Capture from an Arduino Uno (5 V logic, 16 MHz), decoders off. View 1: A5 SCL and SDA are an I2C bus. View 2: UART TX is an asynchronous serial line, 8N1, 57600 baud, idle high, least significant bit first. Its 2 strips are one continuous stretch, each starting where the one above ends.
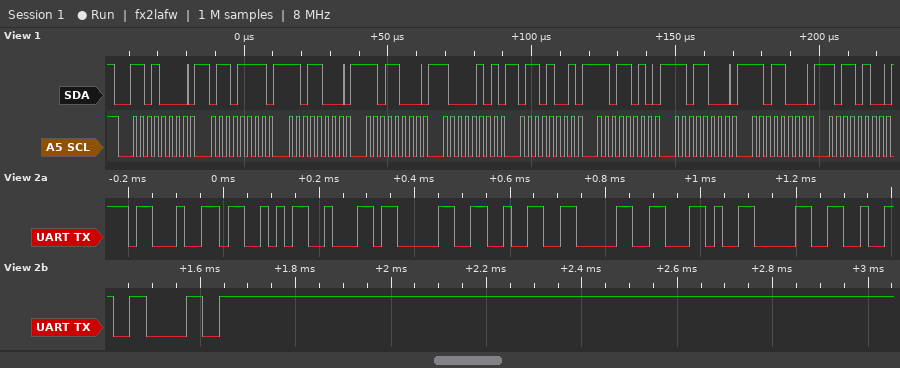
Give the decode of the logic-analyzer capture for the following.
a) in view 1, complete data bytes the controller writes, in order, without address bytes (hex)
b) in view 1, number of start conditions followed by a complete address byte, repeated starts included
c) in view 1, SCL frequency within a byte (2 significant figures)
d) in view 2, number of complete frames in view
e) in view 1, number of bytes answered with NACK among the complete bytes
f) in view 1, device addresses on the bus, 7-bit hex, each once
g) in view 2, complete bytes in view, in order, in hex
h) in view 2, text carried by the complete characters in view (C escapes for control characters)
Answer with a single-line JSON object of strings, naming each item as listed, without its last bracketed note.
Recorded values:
{"in view 1, complete data bytes the controller writes, in order, without address bytes": "6F D8 D8 85 69 DA D8 D8 B4", "in view 1, number of start conditions followed by a complete address byte, repeated starts included": "1", "in view 1, SCL frequency within a byte": "400 kHz", "in view 2, number of complete frames in view": "10", "in view 1, number of bytes answered with NACK among the complete bytes": "0", "in view 1, device addresses on the bus, 7-bit hex, each once": "0x68", "in view 2, complete bytes in view, in order, in hex": "23 53 62 30 32 30 2C 30 32 30", "in view 2, text carried by the complete characters in view": "\"#Sb020,020\""}
